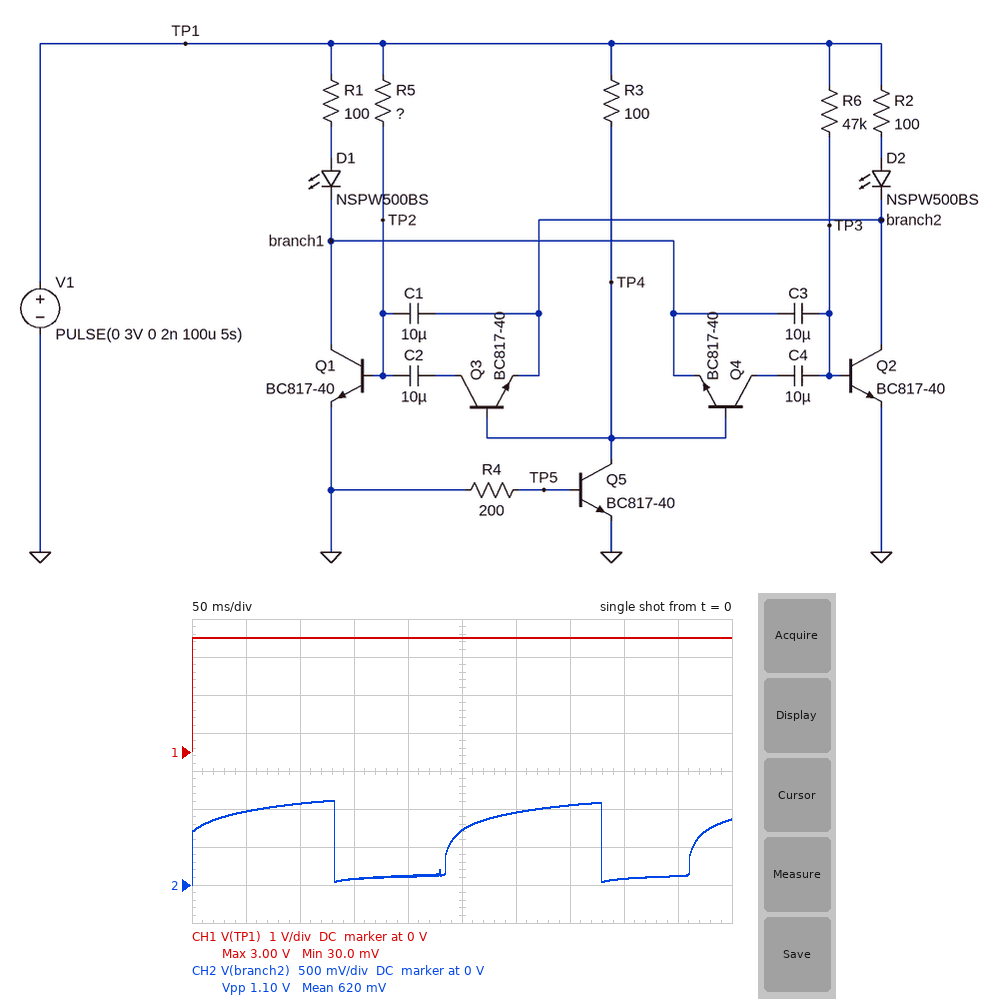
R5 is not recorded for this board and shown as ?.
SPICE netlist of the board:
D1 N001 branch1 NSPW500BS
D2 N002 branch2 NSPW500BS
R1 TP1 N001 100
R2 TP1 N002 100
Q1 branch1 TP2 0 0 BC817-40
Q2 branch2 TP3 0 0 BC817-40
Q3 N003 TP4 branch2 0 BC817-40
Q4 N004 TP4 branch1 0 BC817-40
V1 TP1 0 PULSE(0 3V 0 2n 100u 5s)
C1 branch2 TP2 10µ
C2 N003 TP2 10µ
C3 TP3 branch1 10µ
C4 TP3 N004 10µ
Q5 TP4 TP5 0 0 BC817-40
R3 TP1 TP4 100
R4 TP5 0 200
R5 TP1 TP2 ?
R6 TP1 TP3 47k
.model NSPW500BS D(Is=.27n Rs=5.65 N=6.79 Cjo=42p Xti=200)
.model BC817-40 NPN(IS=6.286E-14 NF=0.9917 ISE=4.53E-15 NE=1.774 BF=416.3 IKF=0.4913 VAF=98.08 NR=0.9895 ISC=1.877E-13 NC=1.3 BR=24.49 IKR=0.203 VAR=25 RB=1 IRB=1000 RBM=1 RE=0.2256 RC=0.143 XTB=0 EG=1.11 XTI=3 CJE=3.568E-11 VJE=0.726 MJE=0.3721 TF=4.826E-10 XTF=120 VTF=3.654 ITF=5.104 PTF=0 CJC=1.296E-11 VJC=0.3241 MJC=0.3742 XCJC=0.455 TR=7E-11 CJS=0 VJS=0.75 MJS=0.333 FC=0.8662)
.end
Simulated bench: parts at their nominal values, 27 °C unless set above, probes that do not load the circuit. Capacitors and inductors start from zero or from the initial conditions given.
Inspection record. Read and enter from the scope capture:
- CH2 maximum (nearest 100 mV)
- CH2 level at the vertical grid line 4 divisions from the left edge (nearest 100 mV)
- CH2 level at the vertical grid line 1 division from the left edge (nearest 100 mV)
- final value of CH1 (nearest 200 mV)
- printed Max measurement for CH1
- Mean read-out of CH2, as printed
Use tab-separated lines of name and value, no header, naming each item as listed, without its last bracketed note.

CH2 maximum	1.1 V
CH2 level at the vertical grid line 4 divisions from the left edge	100 mV
CH2 level at the vertical grid line 1 division from the left edge	1.0 V
final value of CH1	3.0 V
printed Max measurement for CH1	3.00 V
Mean read-out of CH2, as printed	620 mV
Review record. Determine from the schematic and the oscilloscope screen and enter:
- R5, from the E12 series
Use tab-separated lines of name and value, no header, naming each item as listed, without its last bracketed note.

R5, from the E12 series	27 kΩ
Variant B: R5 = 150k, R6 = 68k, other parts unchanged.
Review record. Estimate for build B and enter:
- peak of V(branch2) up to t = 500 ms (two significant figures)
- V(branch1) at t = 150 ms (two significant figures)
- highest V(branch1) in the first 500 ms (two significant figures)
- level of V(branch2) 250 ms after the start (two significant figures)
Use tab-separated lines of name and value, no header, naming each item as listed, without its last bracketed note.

peak of V(branch2) up to t = 500 ms	960 mV
V(branch1) at t = 150 ms	360 mV
highest V(branch1) in the first 500 ms	1.1 V
level of V(branch2) 250 ms after the start	210 mV
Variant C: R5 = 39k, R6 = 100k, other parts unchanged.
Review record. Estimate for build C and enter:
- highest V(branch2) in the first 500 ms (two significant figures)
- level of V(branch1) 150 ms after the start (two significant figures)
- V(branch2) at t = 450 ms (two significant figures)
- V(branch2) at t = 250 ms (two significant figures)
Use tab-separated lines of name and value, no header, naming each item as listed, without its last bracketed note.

highest V(branch2) in the first 500 ms	1.2 V
level of V(branch1) 150 ms after the start	130 mV
V(branch2) at t = 450 ms	1.1 V
V(branch2) at t = 250 ms	100 mV
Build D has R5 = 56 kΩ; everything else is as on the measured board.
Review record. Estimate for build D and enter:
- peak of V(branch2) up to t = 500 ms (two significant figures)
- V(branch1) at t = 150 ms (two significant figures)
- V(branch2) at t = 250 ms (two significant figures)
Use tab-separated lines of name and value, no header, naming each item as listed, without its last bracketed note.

peak of V(branch2) up to t = 500 ms	1.1 V
V(branch1) at t = 150 ms	100 mV
V(branch2) at t = 250 ms	1.1 V
